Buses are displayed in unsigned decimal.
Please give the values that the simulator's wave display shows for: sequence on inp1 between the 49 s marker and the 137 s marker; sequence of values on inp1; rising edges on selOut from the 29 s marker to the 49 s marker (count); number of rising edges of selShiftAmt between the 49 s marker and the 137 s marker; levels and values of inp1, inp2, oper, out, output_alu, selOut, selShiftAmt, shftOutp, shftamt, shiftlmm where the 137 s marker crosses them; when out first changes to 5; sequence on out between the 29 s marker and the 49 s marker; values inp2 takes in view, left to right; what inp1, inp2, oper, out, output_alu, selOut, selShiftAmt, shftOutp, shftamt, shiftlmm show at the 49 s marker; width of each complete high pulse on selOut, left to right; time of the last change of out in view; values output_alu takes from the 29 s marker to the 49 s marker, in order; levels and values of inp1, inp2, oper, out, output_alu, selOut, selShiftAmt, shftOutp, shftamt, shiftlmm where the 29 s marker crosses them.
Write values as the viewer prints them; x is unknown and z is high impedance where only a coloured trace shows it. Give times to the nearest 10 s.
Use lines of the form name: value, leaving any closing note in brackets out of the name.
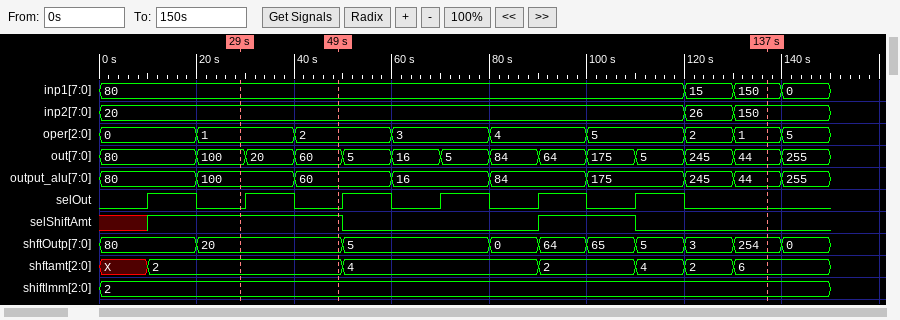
sequence on inp1 between the 49 s marker and the 137 s marker: 80, 15, 150
sequence of values on inp1: 80, 15, 150, 0
rising edges on selOut from the 29 s marker to the 49 s marker: 1
number of rising edges of selShiftAmt between the 49 s marker and the 137 s marker: 1
levels and values of inp1, inp2, oper, out, output_alu, selOut, selShiftAmt, shftOutp, shftamt, shiftlmm where the 137 s marker crosses them: inp1=150, inp2=150, oper=1, out=44, output_alu=44, selOut=0, selShiftAmt=0, shftOutp=254, shftamt=6, shiftlmm=2
when out first changes to 5: 50 s
sequence on out between the 29 s marker and the 49 s marker: 100, 20, 60
values inp2 takes in view, left to right: 20, 26, 150
what inp1, inp2, oper, out, output_alu, selOut, selShiftAmt, shftOutp, shftamt, shiftlmm show at the 49 s marker: inp1=80, inp2=20, oper=2, out=60, output_alu=60, selOut=0, selShiftAmt=1, shftOutp=20, shftamt=2, shiftlmm=2
width of each complete high pulse on selOut, left to right: 10 s, 10 s, 10 s, 10 s, 10 s, 10 s
time of the last change of out in view: 140 s
values output_alu takes from the 29 s marker to the 49 s marker, in order: 100, 60
levels and values of inp1, inp2, oper, out, output_alu, selOut, selShiftAmt, shftOutp, shftamt, shiftlmm where the 29 s marker crosses them: inp1=80, inp2=20, oper=1, out=100, output_alu=100, selOut=0, selShiftAmt=1, shftOutp=20, shftamt=2, shiftlmm=2
